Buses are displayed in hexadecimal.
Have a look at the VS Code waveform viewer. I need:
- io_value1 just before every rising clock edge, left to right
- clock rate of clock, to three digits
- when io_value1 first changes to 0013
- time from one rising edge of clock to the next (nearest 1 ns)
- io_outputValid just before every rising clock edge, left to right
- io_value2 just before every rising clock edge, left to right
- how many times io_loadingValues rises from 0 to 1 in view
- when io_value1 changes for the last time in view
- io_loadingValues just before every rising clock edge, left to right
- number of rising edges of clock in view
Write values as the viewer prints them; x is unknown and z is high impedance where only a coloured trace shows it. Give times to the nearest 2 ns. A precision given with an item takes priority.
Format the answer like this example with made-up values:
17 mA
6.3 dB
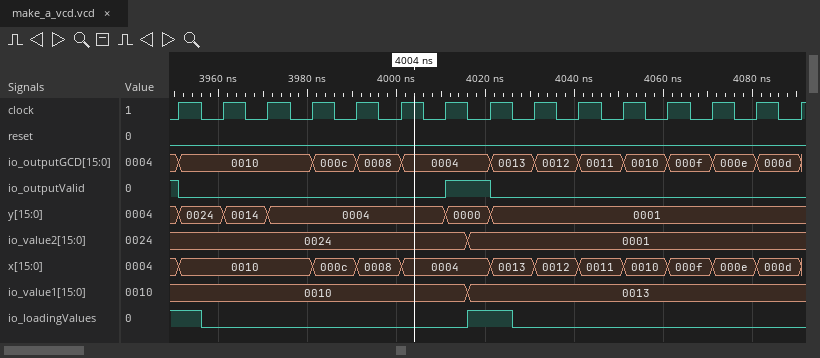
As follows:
0010, 0010, 0010, 0010, 0010, 0010, 0010, 0013, 0013, 0013, 0013, 0013, 0013, 0013, 0013
100 MHz
4016 ns
10 ns
1 0 0 0 0 0 0 1 0 0 0 0 0 0 0
0024, 0024, 0024, 0024, 0024, 0024, 0024, 0001, 0001, 0001, 0001, 0001, 0001, 0001, 0001
1
4016 ns
1 0 0 0 0 0 0 1 0 0 0 0 0 0 0
15
